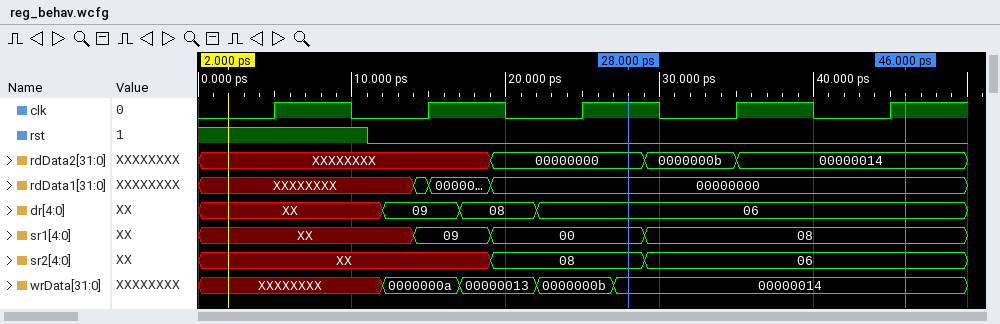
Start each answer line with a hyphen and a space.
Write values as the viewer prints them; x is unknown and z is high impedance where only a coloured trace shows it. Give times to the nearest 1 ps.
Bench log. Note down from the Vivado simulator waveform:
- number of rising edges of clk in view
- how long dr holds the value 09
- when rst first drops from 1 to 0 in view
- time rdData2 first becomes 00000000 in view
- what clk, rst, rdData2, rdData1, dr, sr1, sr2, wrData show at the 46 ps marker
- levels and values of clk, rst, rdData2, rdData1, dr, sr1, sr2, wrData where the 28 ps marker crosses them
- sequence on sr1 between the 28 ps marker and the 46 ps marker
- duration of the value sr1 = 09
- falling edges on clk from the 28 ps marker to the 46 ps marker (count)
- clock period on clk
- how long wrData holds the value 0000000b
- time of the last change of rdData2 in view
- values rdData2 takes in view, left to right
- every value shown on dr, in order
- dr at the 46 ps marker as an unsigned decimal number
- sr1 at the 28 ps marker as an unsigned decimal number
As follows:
- 5
- 5 ps
- 11 ps
- 19 ps
- clk=1, rst=0, rdData2=00000014, rdData1=00000000, dr=06, sr1=08, sr2=06, wrData=00000014
- clk=1, rst=0, rdData2=00000000, rdData1=00000000, dr=06, sr1=00, sr2=08, wrData=00000014
- 00, 08
- 5 ps
- 2
- 10 ps
- 5 ps
- 35 ps
- XXXXXXXX, 00000000, 0000000b, 00000014
- XX, 09, 08, 06
- 6
- 0
